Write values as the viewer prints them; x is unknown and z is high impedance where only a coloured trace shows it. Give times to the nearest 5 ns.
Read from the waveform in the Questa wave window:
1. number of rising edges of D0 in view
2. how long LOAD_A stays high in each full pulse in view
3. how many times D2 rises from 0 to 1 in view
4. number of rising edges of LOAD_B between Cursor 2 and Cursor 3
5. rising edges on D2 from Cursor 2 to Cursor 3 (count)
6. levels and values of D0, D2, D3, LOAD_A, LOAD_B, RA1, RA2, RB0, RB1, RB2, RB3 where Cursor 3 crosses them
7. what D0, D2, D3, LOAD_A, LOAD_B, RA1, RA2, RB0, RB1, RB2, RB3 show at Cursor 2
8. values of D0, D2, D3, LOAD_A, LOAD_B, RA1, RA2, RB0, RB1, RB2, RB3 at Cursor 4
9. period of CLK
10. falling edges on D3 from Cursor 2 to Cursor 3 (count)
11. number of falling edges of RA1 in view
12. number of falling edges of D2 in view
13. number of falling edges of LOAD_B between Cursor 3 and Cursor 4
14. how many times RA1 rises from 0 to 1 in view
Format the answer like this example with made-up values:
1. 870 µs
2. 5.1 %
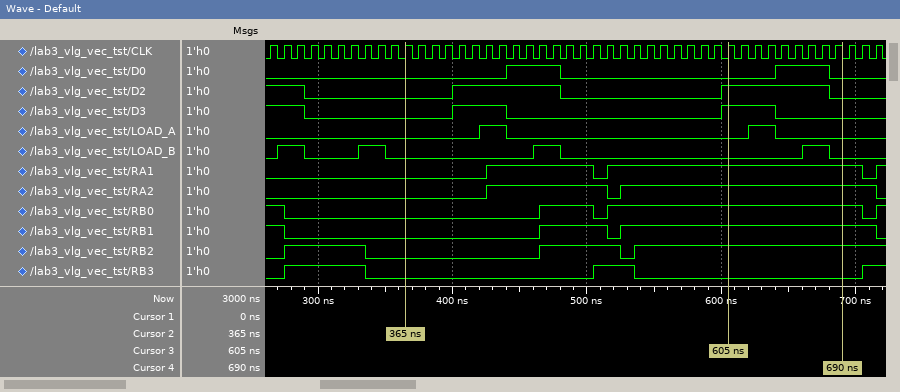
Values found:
1. 2
2. 20 ns, 20 ns
3. 2
4. 1
5. 2
6. D0=0, D2=1, D3=1, LOAD_A=0, LOAD_B=0, RA1=1, RA2=1, RB0=1, RB1=1, RB2=1, RB3=0
7. D0=0, D2=0, D3=0, LOAD_A=0, LOAD_B=0, RA1=0, RA2=0, RB0=0, RB1=0, RB2=0, RB3=0
8. D0=0, D2=0, D3=0, LOAD_A=0, LOAD_B=0, RA1=1, RA2=1, RB0=1, RB1=1, RB2=1, RB3=0
9. 10 ns
10. 1
11. 2
12. 3
13. 1
14. 3
